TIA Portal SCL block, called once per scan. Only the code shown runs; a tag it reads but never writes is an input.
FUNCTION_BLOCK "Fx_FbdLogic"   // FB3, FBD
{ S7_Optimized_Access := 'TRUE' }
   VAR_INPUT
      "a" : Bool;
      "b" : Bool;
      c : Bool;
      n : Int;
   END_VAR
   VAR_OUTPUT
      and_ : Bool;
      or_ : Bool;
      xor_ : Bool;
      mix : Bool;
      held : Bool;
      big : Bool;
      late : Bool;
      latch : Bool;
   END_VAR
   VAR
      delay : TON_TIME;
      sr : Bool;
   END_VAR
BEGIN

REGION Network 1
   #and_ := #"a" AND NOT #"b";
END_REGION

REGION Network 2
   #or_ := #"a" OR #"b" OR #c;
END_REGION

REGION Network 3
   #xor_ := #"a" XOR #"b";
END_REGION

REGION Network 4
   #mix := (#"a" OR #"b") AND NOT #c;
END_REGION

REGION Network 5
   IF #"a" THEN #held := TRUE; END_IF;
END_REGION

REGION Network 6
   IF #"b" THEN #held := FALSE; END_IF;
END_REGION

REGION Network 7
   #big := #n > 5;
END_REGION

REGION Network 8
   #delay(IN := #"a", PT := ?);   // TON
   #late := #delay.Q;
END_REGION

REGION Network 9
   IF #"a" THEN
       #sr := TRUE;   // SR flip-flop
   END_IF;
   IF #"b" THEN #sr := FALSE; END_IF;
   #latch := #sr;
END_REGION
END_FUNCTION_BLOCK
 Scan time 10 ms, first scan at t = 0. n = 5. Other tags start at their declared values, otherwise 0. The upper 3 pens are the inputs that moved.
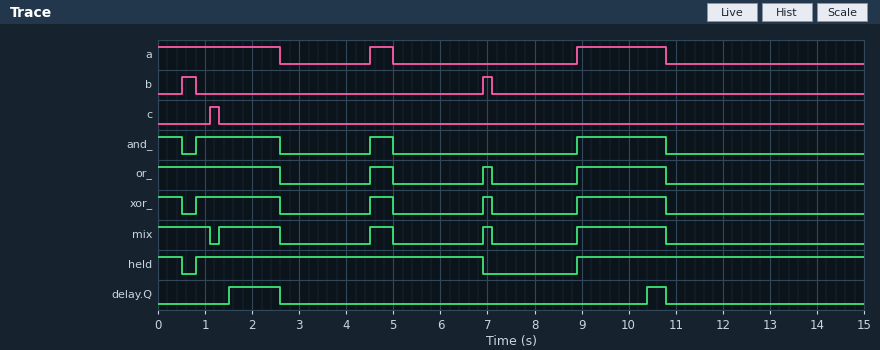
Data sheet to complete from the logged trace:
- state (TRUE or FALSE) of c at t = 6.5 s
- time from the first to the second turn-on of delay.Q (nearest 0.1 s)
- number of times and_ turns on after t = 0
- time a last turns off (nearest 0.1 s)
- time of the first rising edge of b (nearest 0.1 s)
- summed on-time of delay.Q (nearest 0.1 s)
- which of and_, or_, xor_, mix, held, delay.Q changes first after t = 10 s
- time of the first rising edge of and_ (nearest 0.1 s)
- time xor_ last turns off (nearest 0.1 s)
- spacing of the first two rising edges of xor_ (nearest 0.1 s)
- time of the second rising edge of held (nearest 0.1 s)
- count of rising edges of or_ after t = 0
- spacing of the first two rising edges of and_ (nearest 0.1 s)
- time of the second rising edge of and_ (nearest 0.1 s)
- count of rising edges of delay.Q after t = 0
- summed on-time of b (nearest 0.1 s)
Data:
FALSE
8.9 s
3
10.8 s
0.5 s
1.5 s
delay.Q
0.8 s
10.8 s
3.7 s
8.9 s
3
3.7 s
4.5 s
2
0.5 s
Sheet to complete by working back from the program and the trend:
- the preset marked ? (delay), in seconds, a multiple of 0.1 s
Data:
1.5 s
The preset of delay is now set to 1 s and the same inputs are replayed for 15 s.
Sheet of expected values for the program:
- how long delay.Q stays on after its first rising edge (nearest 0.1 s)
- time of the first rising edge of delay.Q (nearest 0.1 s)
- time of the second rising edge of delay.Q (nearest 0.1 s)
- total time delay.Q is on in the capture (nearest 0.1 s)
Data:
1.6 s
1.0 s
9.9 s
2.5 s
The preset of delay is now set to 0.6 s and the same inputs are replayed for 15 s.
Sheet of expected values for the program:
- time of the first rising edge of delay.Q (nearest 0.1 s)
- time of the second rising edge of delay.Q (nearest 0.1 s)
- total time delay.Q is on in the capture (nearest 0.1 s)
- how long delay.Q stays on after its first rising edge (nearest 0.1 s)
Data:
0.6 s
9.5 s
3.3 s
2.0 s
